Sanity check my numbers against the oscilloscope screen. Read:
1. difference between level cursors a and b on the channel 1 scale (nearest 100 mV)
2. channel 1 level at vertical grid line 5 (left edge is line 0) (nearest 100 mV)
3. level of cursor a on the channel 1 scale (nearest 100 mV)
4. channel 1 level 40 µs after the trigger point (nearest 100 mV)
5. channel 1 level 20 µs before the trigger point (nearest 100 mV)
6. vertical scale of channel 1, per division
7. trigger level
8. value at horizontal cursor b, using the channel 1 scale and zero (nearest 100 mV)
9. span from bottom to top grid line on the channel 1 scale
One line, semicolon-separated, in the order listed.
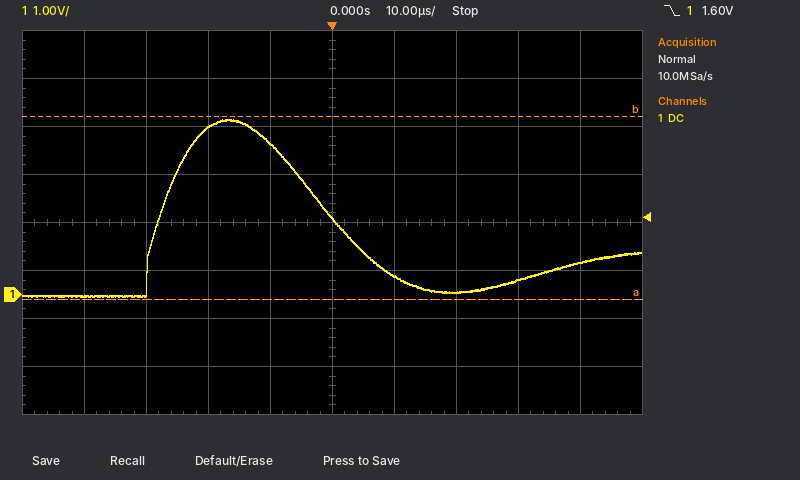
3.8 V; 1.6 V; -100 mV; 700 mV; 3.5 V; 1 V; 1.60 V; 3.7 V; 8 V
